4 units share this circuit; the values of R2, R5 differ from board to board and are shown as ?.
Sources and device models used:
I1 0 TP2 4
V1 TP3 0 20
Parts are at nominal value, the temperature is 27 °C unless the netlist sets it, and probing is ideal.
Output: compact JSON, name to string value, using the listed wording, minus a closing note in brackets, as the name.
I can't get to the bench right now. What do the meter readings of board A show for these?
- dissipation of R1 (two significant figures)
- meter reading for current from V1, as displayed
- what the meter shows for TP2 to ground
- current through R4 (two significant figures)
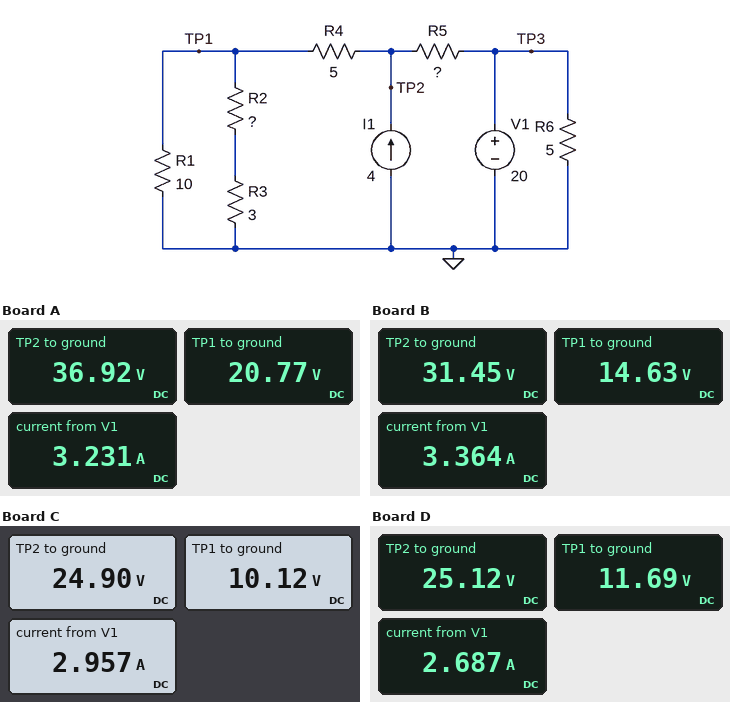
{"dissipation of R1": "43 W", "meter reading for current from V1, as displayed": "3.231 A", "what the meter shows for TP2 to ground": "36.92 V", "current through R4": "3.2 A"}
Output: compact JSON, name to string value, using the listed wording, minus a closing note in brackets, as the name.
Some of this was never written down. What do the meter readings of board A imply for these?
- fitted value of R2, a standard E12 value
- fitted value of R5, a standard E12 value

{"fitted value of R2, a standard E12 value": "15 Ω", "fitted value of R5, a standard E12 value": "22 Ω"}
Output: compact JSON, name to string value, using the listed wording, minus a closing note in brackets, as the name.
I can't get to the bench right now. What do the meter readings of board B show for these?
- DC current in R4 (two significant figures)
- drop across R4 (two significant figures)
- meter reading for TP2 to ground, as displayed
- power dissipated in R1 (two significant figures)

{"DC current in R4": "3.4 A", "drop across R4": "17 V", "meter reading for TP2 to ground, as displayed": "31.45 V", "power dissipated in R1": "21 W"}
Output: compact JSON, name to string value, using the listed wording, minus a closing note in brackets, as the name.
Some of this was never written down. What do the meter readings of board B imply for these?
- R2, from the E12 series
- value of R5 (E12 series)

{"R2, from the E12 series": "4.7 Ω", "value of R5": "18 Ω"}
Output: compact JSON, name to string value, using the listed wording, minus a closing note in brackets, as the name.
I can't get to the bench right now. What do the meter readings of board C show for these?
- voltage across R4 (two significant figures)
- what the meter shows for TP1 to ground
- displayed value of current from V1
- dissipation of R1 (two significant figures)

{"voltage across R4": "15 V", "what the meter shows for TP1 to ground": "10.12 V", "displayed value of current from V1": "2.957 A", "dissipation of R1": "10 W"}
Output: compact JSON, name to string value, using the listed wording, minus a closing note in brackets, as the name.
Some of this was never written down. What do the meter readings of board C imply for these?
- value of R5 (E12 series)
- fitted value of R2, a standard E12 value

{"value of R5": "4.7 Ω", "fitted value of R2, a standard E12 value": "2.2 Ω"}
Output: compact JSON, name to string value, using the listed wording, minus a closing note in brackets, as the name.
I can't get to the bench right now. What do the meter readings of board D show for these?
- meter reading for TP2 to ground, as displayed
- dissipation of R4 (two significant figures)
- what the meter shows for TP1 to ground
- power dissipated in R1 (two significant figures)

{"meter reading for TP2 to ground, as displayed": "25.12 V", "dissipation of R4": "36 W", "what the meter shows for TP1 to ground": "11.69 V", "power dissipated in R1": "14 W"}
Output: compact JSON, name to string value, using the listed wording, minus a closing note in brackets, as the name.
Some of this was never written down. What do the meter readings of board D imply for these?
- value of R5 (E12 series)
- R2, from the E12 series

{"value of R5": "3.9 Ω", "R2, from the E12 series": "4.7 Ω"}
